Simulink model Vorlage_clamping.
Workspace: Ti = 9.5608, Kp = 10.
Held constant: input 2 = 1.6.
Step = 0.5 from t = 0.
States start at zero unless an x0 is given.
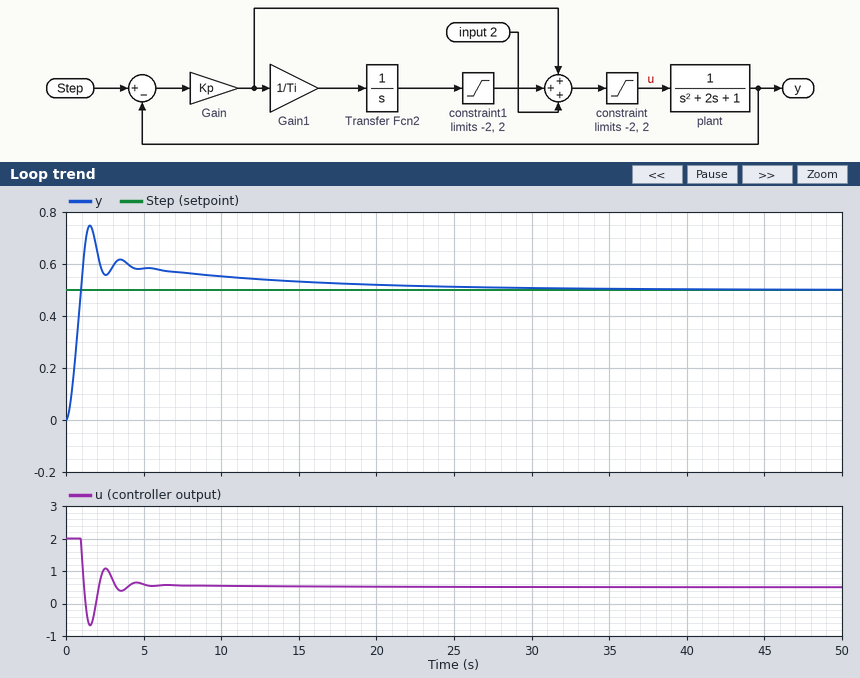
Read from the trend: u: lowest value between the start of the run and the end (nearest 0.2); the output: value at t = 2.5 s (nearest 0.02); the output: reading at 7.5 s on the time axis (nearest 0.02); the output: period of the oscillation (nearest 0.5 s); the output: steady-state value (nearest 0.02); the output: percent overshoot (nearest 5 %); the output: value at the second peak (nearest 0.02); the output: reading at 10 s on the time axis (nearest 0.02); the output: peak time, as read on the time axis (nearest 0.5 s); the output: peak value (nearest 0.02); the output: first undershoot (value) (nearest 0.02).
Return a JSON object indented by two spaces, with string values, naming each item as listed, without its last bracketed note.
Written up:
{
  "u: lowest value between the start of the run and the end": "-0.6",
  "the output: value at t = 2.5 s": "0.56",
  "the output: reading at 7.5 s on the time axis": "0.56",
  "the output: period of the oscillation": "2.0 s",
  "the output: steady-state value": "0.50",
  "the output: percent overshoot": "50 %",
  "the output: value at the second peak": "0.62",
  "the output: reading at 10 s on the time axis": "0.56",
  "the output: peak time, as read on the time axis": "1.5 s",
  "the output: peak value": "0.74",
  "the output: first undershoot (value)": "0.56"
}
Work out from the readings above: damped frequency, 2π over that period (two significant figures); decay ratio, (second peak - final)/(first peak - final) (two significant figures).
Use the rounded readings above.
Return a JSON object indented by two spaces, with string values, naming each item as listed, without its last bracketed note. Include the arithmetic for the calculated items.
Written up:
{
  "damped frequency, 2π over that period": "2π / 2 = 3.1 rad/s",
  "decay ratio, (second peak - final)/(first peak - final)": "(0.62 - 0.5) / (0.74 - 0.5) = 0.50"
}
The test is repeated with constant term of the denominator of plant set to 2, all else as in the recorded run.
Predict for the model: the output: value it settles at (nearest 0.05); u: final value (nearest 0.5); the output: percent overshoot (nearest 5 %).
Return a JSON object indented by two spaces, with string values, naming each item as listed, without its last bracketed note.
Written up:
{
  "the output: value it settles at": "0.50",
  "u: final value": "1.0",
  "the output: percent overshoot": "35 %"
}
